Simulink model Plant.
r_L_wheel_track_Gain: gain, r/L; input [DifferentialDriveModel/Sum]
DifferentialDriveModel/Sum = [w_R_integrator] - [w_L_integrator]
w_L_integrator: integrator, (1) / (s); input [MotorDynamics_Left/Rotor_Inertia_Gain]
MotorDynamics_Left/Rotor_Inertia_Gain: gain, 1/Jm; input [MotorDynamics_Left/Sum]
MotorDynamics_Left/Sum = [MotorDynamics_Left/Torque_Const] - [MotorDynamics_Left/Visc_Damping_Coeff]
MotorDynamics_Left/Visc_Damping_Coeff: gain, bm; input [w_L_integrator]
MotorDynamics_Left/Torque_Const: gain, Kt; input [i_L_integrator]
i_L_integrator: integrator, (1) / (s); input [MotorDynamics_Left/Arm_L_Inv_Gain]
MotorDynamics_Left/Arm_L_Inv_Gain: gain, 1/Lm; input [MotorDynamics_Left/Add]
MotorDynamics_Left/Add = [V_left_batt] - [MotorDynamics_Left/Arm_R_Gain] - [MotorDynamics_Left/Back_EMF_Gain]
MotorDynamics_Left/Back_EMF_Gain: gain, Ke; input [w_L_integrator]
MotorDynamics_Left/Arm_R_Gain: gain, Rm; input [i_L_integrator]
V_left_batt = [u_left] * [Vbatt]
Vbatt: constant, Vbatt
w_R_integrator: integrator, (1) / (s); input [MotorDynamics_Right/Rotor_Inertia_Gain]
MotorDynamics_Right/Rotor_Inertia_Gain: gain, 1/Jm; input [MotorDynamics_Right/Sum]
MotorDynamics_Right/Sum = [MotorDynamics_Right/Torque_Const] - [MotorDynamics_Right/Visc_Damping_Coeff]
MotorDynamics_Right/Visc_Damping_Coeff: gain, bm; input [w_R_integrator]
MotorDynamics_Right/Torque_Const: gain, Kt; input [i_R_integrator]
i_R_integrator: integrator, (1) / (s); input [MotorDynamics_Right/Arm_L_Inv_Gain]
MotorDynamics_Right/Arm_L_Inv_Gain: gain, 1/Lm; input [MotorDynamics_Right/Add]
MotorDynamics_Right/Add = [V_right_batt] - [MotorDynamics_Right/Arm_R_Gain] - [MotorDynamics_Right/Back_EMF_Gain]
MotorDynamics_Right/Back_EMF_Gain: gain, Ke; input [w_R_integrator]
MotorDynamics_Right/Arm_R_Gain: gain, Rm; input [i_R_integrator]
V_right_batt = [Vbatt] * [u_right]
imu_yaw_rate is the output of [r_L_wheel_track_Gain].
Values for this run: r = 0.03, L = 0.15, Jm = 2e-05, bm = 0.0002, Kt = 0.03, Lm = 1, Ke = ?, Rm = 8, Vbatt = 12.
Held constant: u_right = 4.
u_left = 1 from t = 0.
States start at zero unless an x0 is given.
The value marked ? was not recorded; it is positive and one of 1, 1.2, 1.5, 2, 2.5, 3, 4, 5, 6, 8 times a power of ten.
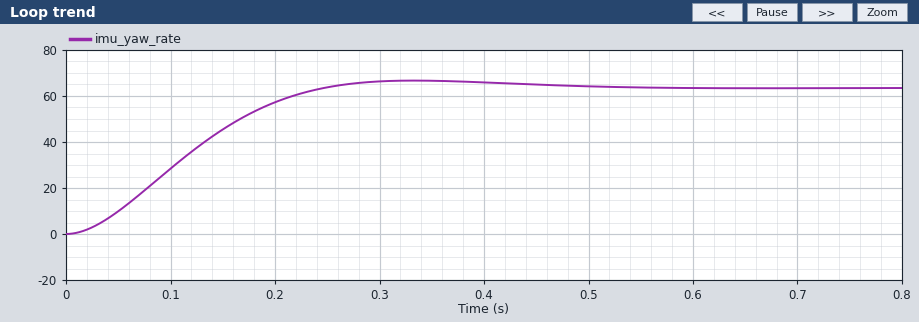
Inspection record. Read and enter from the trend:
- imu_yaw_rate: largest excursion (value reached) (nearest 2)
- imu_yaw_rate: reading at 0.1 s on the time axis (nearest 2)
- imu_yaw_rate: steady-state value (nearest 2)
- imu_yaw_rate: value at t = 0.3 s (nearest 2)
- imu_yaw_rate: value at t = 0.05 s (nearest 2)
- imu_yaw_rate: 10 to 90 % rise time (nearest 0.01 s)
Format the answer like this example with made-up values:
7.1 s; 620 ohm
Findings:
66; 28; 64; 66; 10; 0.16 s
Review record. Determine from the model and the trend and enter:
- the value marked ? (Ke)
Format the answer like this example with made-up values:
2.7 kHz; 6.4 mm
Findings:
0.06
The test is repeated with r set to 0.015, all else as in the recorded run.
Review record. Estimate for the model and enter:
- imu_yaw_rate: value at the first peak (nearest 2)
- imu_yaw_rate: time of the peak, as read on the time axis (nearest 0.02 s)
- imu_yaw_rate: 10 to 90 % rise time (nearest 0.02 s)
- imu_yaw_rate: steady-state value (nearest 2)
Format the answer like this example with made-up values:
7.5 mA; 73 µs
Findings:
34; 0.34 s; 0.16 s; 32
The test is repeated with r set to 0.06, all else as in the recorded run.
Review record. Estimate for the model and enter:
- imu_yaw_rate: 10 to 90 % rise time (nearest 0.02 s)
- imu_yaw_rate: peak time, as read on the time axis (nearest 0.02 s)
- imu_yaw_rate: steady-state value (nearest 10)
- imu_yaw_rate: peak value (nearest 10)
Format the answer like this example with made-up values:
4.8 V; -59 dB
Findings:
0.16 s; 0.34 s; 130; 130
